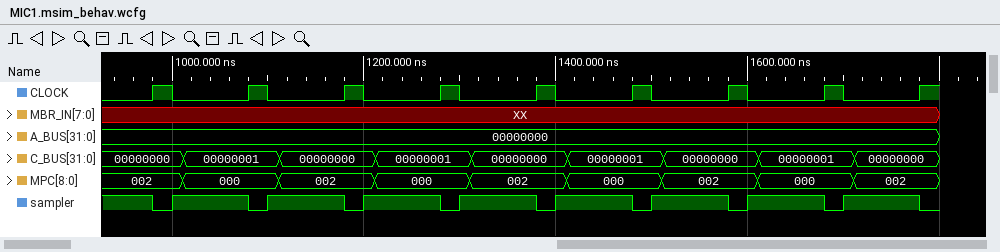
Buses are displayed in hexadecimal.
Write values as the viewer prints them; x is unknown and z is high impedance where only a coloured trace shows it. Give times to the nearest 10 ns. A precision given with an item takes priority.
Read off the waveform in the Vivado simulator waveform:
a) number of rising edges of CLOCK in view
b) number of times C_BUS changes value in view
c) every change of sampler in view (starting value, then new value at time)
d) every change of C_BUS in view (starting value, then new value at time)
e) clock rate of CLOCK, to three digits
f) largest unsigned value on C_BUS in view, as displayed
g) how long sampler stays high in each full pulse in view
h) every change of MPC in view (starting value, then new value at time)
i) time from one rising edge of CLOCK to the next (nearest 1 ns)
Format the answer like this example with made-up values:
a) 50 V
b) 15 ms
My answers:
a) 9
b) 8
c) 1, 0 at 980 ns, 1 at 1000 ns, 0 at 1080 ns, 1 at 1100 ns, 0 at 1180 ns, 1 at 1200 ns, 0 at 1280 ns, 1 at 1300 ns, 0 at 1380 ns, 1 at 1400 ns, 0 at 1480 ns, 1 at 1500 ns, 0 at 1580 ns, 1 at 1600 ns, 0 at 1680 ns, 1 at 1700 ns, 0 at 1780 ns
d) 00000000, 00000001 at 1010 ns, 00000000 at 1110 ns, 00000001 at 1210 ns, 00000000 at 1310 ns, 00000001 at 1410 ns, 00000000 at 1510 ns, 00000001 at 1610 ns, 00000000 at 1710 ns
e) 10.0 MHz
f) 00000001
g) 80 ns, 80 ns, 80 ns, 80 ns, 80 ns, 80 ns, 80 ns, 80 ns
h) 002, 000 at 1010 ns, 002 at 1110 ns, 000 at 1210 ns, 002 at 1310 ns, 000 at 1410 ns, 002 at 1510 ns, 000 at 1610 ns, 002 at 1710 ns
i) 100 ns
